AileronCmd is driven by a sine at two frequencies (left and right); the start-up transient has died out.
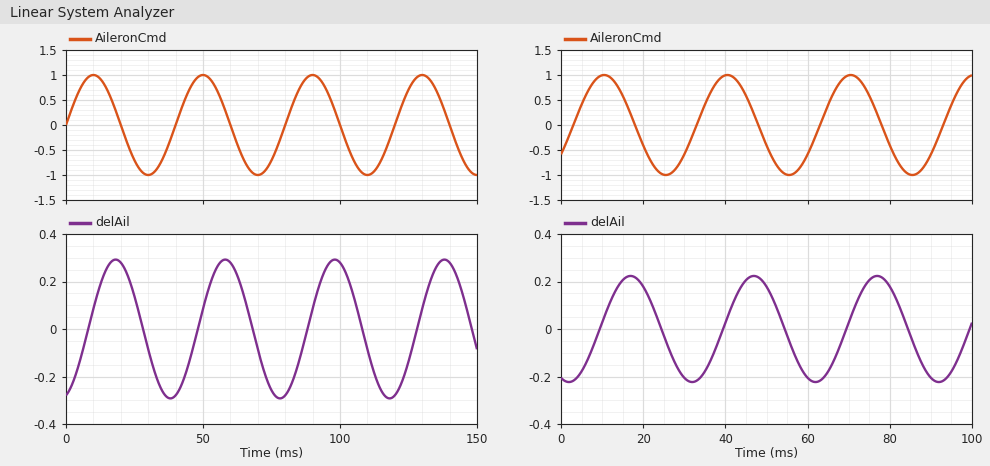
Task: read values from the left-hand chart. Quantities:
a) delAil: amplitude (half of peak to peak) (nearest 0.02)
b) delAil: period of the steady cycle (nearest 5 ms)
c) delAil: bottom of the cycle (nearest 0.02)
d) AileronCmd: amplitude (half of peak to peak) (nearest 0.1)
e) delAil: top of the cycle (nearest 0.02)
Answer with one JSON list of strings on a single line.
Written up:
["0.30", "40 ms", "-0.30", "1.0", "0.30"]
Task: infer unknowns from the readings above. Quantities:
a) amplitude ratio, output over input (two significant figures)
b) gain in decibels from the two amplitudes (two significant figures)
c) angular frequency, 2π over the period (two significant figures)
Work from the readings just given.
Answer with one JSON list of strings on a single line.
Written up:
["0.30", "-10 dB", "0.16 rad/ms"]
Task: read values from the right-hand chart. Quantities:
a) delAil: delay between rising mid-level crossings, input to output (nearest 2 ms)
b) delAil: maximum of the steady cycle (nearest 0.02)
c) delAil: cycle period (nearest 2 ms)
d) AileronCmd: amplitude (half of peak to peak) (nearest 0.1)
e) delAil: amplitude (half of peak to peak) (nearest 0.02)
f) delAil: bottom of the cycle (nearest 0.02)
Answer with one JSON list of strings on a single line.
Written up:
["6 ms", "0.22", "30 ms", "1.0", "0.22", "-0.22"]
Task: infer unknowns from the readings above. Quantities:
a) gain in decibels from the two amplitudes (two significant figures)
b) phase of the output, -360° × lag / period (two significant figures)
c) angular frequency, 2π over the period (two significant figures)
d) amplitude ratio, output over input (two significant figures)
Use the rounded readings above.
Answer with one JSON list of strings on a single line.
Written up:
["-13 dB", "-72°", "0.21 rad/ms", "0.22"]
